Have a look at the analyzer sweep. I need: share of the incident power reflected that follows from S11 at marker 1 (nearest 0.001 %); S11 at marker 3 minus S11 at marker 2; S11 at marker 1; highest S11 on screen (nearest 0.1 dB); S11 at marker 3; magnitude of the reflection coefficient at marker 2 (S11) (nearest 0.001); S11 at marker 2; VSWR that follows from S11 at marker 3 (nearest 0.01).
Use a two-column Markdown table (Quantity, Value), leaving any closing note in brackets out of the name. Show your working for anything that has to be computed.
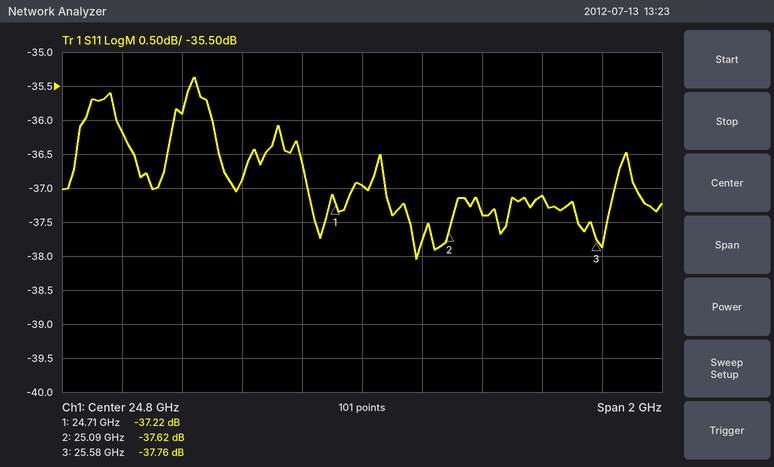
| Quantity | Value |
|---|---|
| share of the incident power reflected that follows from S11 at marker 1 | 10^(-37.22/10) ≈ 0.019 % |
| S11 at marker 3 minus S11 at marker 2 | -37.76 − (-37.62) = -0.14 dB |
| S11 at marker 1 | -37.22 dB |
| highest S11 on screen | -35.4 dB |
| S11 at marker 3 | -37.76 dB |
| magnitude of the reflection coefficient at marker 2 (S11) | 10^(-37.62/20) ≈ 0.013 |
| S11 at marker 2 | -37.62 dB |
| VSWR that follows from S11 at marker 3 | (1 + 0.0129)/(1 − 0.0129) ≈ 1.03 |
